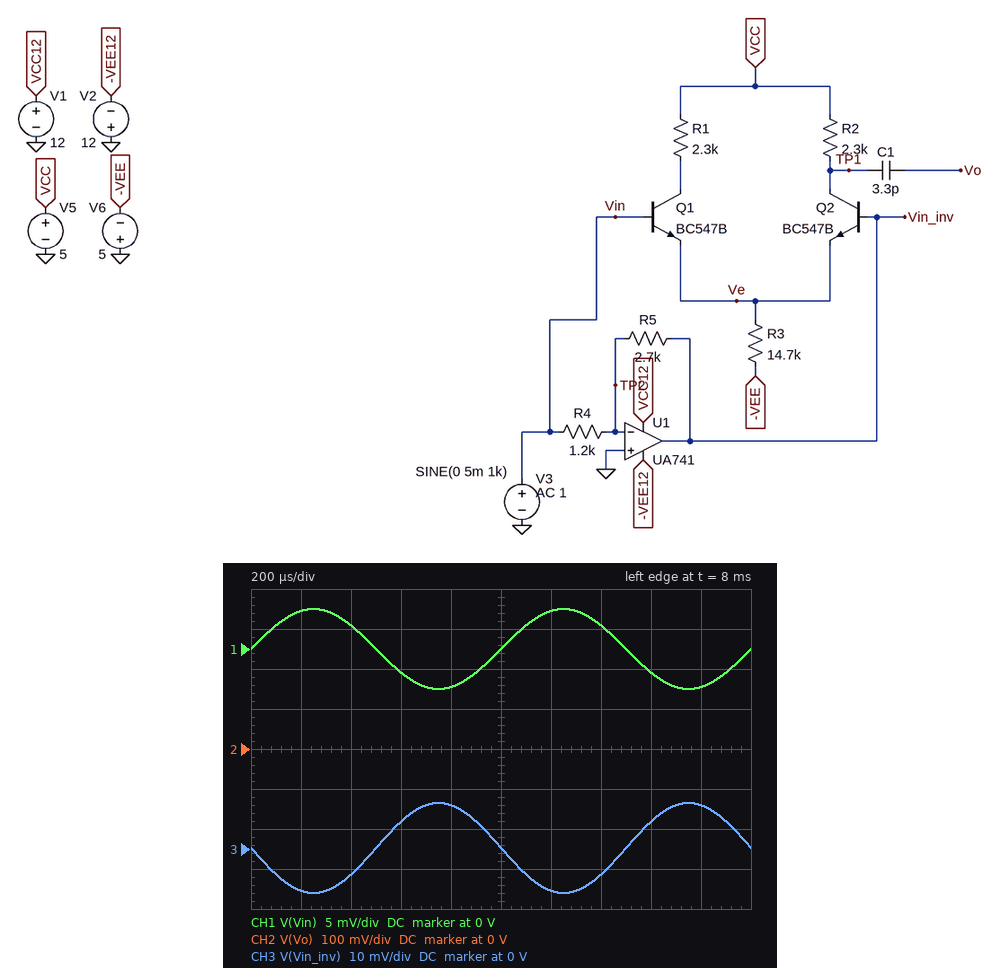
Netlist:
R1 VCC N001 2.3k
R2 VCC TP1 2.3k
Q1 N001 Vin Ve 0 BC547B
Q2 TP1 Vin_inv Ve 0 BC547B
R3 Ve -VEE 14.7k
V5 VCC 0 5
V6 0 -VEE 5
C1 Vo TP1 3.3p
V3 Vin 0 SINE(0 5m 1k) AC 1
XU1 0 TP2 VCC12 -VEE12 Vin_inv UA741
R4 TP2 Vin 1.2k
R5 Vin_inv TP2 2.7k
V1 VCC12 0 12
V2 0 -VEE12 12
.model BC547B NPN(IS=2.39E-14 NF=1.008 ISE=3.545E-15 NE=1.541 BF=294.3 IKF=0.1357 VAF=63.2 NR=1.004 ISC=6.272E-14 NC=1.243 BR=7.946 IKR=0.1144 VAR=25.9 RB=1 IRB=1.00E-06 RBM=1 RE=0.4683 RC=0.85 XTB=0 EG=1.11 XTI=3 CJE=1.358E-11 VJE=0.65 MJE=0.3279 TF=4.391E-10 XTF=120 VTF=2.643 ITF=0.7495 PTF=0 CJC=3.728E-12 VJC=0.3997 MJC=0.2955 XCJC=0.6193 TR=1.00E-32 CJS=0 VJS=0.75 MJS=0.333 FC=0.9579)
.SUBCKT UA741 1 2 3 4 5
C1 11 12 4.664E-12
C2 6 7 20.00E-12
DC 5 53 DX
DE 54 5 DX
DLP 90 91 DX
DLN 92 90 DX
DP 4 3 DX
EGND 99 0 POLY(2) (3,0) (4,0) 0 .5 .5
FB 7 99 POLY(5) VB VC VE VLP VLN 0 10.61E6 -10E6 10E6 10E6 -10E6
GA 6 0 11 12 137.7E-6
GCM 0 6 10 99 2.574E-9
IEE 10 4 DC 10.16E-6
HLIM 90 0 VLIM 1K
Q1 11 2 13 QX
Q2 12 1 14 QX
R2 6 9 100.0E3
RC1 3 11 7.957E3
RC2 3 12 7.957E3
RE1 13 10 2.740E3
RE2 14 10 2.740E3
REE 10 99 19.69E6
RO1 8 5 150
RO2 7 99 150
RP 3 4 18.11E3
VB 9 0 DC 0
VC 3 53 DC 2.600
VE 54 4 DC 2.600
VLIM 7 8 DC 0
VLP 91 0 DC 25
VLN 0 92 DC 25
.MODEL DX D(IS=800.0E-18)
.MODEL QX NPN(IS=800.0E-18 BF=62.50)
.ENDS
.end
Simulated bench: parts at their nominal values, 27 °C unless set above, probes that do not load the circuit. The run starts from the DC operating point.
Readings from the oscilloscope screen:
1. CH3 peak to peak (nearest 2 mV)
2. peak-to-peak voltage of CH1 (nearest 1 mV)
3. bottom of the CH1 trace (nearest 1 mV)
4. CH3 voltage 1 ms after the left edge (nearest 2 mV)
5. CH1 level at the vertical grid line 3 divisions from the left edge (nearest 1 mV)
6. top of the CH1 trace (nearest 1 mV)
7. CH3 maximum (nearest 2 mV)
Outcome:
22 mV
10 mV
-5 mV
0 V
-3 mV
5 mV
12 mV
